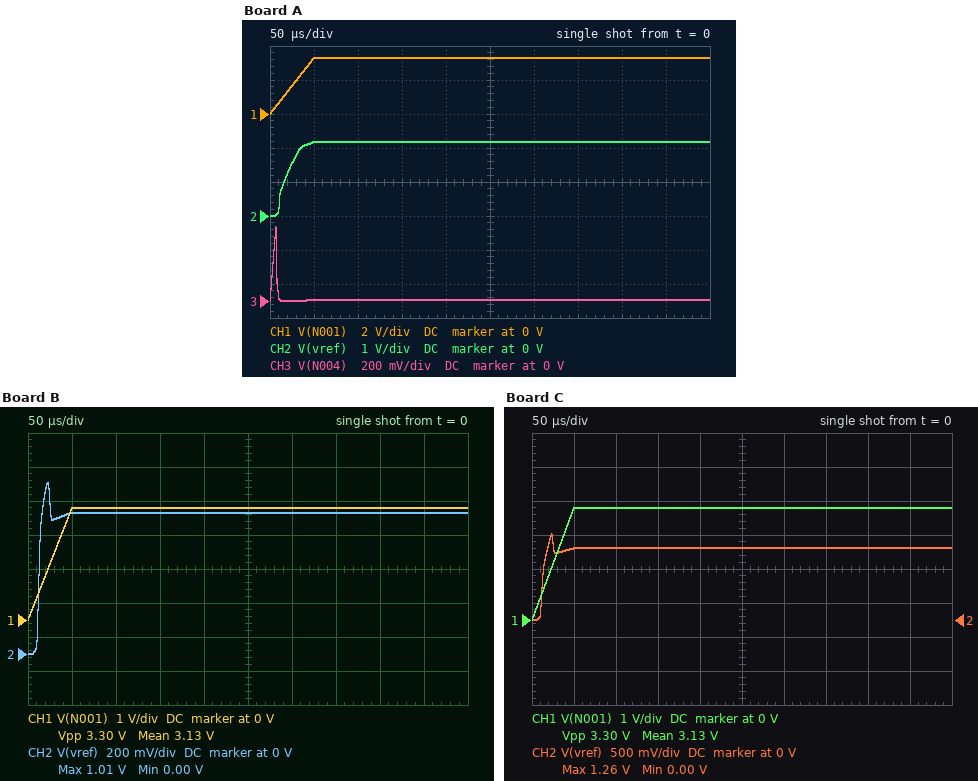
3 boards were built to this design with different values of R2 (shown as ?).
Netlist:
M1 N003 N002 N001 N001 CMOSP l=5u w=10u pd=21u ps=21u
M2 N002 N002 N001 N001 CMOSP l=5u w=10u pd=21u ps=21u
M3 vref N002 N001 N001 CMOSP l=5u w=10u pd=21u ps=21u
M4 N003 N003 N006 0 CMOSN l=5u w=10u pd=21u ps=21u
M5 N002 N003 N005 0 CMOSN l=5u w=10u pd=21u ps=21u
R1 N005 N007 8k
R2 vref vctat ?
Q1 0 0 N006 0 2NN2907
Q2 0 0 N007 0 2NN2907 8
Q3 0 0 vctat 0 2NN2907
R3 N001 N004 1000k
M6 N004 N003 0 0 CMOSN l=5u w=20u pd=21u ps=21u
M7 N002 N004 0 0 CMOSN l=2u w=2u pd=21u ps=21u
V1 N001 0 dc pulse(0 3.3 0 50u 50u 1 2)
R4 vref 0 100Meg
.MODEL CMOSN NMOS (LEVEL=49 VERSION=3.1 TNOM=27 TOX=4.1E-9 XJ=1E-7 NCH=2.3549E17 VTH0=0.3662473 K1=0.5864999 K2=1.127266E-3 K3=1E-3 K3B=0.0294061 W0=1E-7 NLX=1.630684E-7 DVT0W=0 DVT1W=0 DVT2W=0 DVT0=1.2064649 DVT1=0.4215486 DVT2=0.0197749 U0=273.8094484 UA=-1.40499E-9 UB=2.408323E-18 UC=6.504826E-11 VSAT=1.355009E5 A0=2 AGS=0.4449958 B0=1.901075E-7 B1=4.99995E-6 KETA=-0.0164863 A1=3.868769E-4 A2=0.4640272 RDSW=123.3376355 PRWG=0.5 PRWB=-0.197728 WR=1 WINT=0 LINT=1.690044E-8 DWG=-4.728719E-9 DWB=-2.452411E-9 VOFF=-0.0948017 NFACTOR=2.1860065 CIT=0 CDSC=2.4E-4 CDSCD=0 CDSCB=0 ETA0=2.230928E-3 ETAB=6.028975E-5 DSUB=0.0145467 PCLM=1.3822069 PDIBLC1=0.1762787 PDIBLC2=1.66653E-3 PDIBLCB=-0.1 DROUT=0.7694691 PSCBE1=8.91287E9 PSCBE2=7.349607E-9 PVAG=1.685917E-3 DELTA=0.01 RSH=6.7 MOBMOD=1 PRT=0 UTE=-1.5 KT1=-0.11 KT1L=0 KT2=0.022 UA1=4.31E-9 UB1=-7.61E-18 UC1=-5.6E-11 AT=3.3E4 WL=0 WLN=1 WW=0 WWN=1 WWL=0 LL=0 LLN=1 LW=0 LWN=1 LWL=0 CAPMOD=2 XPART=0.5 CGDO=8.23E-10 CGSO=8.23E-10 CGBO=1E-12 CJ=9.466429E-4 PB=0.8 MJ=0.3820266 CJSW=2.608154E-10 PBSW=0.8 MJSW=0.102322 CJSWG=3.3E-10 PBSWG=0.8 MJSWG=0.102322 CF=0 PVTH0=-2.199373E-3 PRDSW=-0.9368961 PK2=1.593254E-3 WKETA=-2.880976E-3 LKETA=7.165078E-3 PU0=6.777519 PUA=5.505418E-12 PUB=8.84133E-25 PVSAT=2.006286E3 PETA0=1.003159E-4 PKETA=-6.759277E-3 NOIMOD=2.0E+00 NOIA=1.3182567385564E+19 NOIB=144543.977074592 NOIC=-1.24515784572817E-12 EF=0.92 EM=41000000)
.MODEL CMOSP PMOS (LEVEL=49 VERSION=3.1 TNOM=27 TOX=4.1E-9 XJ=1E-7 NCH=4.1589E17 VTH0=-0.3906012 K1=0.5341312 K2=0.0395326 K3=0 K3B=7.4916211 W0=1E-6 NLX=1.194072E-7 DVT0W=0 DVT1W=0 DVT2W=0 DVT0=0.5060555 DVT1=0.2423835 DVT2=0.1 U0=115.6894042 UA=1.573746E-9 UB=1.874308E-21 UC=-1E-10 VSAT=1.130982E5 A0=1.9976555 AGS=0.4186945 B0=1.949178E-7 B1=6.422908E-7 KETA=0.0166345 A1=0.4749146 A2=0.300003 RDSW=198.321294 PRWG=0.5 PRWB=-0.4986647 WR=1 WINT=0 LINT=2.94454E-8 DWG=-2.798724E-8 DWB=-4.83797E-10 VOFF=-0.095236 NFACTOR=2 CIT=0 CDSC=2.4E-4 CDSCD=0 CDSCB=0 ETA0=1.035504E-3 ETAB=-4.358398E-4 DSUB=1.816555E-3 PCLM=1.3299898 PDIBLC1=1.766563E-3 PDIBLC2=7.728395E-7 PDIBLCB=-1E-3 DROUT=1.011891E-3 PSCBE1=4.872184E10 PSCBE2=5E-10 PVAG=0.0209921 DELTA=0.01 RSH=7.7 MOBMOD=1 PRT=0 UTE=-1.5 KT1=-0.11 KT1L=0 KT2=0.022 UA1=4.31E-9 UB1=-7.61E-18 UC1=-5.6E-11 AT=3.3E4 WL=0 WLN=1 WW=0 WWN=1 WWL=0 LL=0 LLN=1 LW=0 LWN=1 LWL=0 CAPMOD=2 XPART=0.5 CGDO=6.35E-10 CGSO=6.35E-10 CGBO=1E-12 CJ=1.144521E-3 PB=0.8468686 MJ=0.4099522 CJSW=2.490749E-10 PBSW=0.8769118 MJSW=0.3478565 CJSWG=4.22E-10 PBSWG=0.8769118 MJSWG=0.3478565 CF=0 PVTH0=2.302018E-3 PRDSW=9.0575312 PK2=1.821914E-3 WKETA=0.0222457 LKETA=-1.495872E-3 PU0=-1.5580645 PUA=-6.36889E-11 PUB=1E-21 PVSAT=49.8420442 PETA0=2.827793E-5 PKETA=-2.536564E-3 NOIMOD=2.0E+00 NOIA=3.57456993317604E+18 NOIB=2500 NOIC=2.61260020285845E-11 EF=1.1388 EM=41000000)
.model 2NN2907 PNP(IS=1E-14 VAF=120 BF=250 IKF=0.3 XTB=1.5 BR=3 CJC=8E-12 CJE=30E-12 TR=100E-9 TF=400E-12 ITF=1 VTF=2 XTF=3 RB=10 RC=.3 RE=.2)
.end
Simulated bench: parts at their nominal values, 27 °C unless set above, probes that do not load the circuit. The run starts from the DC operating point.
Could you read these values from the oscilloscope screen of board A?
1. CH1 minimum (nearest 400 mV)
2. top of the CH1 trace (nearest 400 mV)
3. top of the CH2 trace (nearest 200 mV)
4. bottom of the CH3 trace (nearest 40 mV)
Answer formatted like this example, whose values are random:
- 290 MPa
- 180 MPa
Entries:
- 0 V
- 3.2 V
- 2.2 V
- 0 V
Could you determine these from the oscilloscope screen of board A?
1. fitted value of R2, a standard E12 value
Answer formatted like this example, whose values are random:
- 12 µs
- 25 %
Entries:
- 220 kΩ
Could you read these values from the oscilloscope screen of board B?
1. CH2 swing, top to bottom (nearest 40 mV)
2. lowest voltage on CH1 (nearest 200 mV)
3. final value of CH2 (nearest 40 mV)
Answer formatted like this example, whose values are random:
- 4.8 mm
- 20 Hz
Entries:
- 1.00 V
- 0 V
- 840 mV
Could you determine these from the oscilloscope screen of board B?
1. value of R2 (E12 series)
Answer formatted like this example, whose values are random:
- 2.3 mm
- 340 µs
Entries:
- 39 kΩ
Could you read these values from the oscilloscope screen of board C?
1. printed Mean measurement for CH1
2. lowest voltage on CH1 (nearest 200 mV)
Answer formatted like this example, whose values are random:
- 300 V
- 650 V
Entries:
- 3.13 V
- 0 V
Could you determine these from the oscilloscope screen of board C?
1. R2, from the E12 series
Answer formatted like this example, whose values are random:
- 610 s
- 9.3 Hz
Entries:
- 68 kΩ
